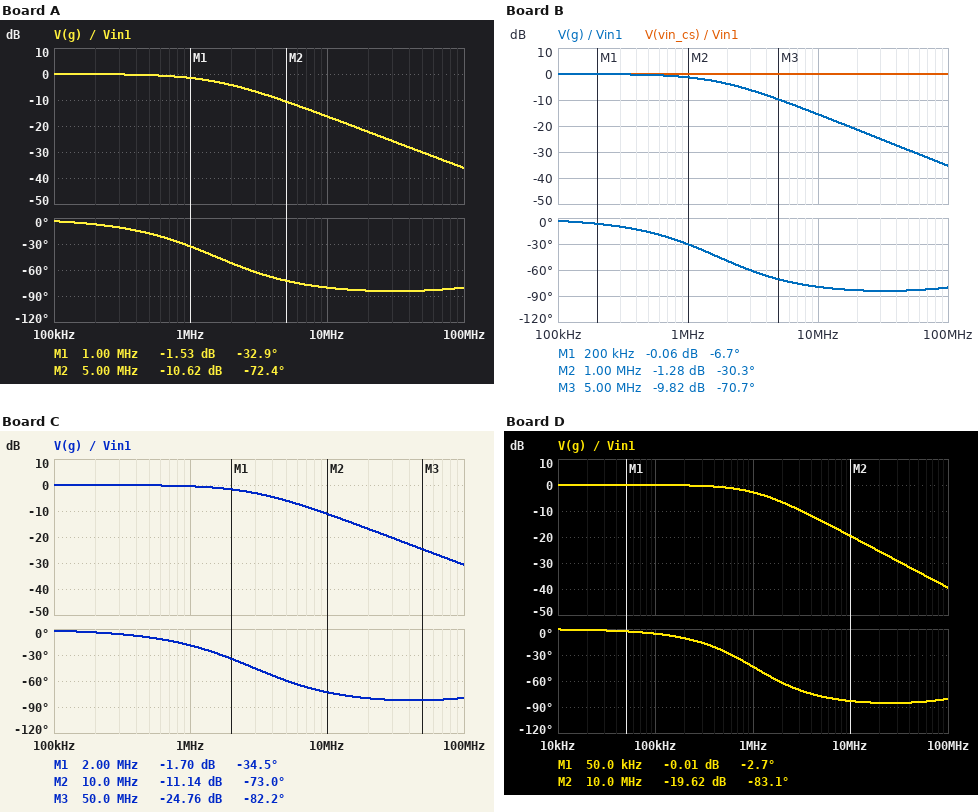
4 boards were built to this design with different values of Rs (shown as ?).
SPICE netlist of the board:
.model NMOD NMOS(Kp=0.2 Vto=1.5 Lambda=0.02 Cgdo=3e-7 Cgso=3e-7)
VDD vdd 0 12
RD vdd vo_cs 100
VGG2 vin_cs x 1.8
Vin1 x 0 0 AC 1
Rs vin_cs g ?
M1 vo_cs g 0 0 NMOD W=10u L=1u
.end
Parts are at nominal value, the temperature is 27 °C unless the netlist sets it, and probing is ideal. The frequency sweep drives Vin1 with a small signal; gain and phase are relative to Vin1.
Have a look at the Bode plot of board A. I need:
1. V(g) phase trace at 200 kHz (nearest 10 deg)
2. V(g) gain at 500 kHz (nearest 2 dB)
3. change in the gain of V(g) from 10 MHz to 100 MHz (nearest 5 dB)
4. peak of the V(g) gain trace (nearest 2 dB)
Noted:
-10 deg
0 dB
-20 dB
0 dB
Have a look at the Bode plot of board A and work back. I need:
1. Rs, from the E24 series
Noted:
620 Ω
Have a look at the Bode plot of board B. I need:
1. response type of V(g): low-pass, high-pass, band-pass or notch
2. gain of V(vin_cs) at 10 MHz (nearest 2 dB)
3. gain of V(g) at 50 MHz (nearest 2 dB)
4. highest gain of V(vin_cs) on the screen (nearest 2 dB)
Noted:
low-pass
0 dB
-30 dB
0 dB
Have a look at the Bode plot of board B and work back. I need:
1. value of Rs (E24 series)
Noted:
560 Ω
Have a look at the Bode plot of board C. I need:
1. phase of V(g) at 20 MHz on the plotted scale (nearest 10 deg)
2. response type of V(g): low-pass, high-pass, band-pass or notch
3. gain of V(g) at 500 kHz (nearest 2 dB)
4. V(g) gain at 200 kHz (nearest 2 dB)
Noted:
-80 deg
low-pass
0 dB
0 dB
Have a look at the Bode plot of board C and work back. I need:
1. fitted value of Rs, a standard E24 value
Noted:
330 Ω
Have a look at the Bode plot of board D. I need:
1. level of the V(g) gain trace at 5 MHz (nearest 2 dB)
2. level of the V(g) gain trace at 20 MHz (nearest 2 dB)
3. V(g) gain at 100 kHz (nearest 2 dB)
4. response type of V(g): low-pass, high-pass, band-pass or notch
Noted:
-14 dB
-26 dB
0 dB
low-pass
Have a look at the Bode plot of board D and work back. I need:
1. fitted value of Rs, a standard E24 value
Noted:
910 Ω
